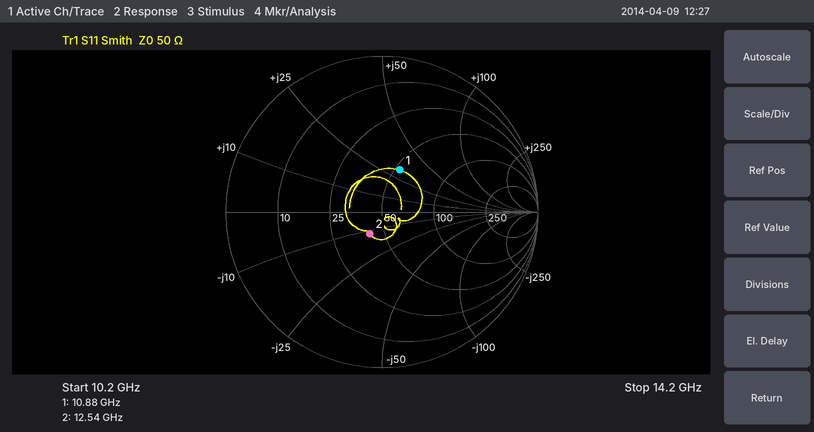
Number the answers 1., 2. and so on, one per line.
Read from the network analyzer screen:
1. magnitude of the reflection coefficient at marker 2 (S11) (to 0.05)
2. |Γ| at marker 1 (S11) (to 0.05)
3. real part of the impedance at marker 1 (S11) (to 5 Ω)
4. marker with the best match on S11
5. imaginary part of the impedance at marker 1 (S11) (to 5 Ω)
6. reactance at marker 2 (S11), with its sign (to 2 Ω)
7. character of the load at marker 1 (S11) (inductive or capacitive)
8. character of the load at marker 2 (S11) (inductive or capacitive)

1. 0.15
2. 0.30
3. 55 Ω
4. marker 2
5. +30 Ω
6. -12 Ω
7. inductive
8. capacitive
